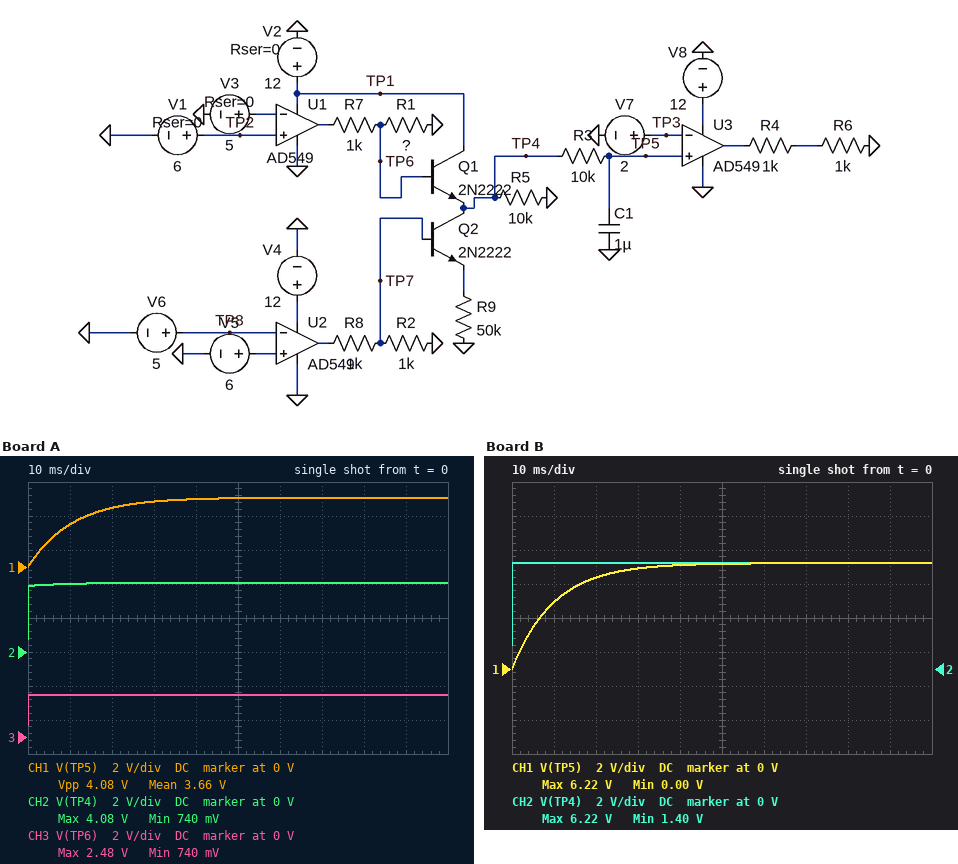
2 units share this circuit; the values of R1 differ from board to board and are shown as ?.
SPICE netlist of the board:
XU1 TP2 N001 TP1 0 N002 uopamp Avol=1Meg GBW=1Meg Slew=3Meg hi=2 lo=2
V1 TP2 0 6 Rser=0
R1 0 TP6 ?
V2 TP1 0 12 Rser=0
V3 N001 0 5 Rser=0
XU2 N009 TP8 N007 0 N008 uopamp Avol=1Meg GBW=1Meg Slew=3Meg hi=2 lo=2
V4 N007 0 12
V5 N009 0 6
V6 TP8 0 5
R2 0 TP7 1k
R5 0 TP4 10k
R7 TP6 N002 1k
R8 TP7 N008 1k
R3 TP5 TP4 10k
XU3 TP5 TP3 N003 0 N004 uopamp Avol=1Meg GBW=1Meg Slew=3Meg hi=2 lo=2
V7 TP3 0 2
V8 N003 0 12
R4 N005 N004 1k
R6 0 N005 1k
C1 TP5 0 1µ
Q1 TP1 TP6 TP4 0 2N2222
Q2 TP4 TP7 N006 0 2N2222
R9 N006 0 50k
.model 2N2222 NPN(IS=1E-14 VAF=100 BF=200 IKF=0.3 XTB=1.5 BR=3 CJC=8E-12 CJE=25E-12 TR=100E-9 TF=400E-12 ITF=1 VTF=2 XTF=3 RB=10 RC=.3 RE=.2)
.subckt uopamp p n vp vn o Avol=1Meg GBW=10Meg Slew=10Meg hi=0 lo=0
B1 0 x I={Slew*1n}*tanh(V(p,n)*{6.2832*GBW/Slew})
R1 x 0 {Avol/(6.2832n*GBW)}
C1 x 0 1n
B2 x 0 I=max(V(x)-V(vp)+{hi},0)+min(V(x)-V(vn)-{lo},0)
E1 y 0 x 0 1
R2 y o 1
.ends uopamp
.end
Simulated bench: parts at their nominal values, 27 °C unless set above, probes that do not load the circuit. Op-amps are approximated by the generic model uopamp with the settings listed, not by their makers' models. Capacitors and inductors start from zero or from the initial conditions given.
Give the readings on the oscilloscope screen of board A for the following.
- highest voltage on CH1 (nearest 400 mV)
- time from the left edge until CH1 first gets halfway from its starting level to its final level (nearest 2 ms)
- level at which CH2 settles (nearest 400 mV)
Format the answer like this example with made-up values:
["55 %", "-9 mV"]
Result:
["4.0 V", "8 ms", "4.0 V"]
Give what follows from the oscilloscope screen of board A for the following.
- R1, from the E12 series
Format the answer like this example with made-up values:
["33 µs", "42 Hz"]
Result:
["330 Ω"]
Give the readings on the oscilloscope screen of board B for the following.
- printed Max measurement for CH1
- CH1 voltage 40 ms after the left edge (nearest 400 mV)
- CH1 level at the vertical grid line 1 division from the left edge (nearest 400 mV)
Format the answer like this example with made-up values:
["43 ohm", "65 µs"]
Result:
["6.22 V", "6.0 V", "4.0 V"]
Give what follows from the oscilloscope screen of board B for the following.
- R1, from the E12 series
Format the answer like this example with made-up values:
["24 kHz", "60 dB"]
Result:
["2.2 kΩ"]
